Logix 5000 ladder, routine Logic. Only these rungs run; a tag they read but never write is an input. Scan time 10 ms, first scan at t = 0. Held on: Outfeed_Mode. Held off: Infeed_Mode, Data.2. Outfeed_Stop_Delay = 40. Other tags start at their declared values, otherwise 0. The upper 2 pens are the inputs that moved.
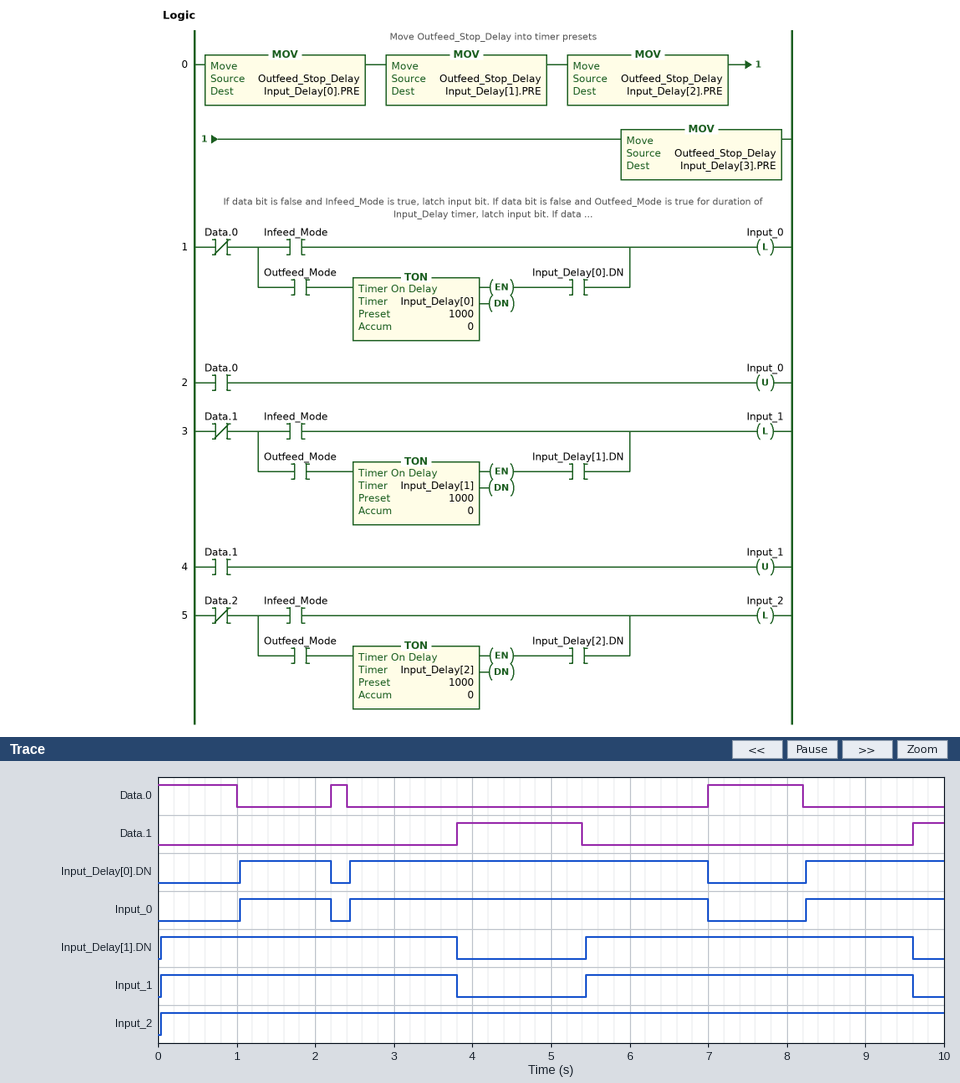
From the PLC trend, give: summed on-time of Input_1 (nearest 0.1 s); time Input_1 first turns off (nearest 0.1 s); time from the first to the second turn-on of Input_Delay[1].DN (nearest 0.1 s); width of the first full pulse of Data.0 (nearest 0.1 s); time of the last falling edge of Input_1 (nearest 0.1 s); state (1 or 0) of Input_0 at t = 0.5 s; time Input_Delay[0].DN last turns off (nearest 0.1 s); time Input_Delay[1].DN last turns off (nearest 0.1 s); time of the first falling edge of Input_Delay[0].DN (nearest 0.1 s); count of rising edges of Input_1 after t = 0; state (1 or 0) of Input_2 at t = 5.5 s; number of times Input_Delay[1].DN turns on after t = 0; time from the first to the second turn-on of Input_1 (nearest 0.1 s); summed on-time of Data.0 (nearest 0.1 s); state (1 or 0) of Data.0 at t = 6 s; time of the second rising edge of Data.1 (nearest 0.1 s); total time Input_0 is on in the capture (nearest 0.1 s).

7.9 s
3.8 s
5.4 s
0.2 s
9.6 s
0
7.0 s
9.6 s
2.2 s
2
1
2
5.4 s
2.4 s
0
9.6 s
7.5 s
